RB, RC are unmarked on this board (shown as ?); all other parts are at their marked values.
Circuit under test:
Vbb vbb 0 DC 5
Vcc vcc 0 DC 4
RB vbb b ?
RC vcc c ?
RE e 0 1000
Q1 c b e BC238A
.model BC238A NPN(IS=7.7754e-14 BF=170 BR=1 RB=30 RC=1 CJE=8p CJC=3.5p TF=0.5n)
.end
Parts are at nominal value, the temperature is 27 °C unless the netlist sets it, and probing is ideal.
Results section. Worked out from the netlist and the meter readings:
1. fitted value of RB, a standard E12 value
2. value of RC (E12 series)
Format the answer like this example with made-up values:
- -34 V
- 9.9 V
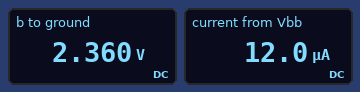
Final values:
- 220 kΩ
- 1.2 kΩ
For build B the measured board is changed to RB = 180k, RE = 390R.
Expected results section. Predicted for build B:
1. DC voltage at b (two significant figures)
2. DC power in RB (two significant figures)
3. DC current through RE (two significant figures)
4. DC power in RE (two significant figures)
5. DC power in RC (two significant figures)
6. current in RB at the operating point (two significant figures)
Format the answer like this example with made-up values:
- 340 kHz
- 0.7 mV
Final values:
- 1.6 V
- 65 µW
- 2.4 mA
- 2.3 mW
- 7.0 mW
- 19 µA
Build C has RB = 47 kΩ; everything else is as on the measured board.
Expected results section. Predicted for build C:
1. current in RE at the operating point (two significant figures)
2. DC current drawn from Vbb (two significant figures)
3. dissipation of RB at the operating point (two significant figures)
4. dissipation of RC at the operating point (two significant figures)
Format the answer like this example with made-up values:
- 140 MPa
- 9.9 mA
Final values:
- 1.8 mA
- 55 µA
- 140 µW
- 3.7 mW
